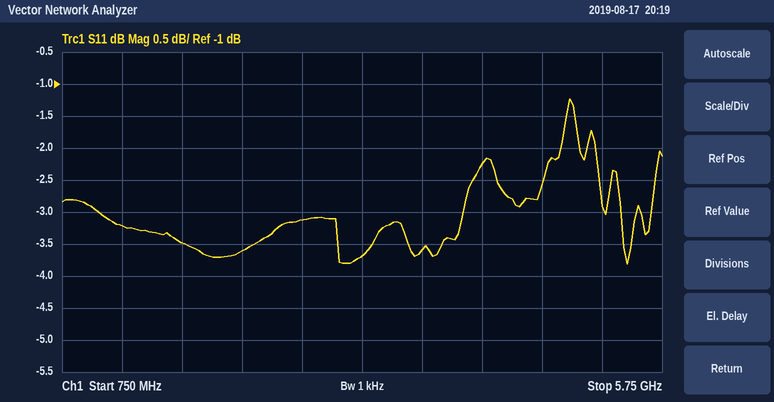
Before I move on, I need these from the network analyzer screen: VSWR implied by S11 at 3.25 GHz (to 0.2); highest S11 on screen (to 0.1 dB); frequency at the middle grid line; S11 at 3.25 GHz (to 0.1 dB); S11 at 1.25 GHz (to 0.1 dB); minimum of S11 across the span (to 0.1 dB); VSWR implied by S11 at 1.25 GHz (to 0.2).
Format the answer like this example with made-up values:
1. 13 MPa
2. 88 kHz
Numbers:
1. 4.8
2. -1.2 dB
3. 3.25 GHz
4. -3.7 dB
5. -3.2 dB
6. -3.8 dB
7. 5.4
